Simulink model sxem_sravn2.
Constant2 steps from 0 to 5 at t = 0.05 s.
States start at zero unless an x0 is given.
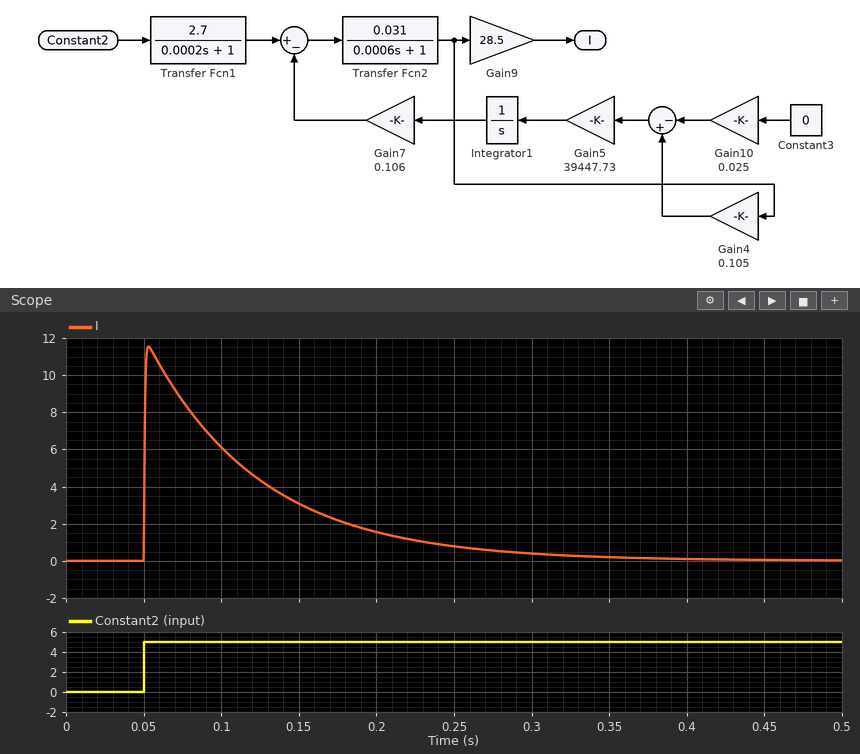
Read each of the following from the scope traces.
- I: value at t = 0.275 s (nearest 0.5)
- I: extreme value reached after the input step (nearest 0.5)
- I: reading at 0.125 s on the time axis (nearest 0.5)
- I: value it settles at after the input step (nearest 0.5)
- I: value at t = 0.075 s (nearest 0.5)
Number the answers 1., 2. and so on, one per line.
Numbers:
1. 0.5
2. 11.5
3. 4.5
4. 0.0
5. 8.5
